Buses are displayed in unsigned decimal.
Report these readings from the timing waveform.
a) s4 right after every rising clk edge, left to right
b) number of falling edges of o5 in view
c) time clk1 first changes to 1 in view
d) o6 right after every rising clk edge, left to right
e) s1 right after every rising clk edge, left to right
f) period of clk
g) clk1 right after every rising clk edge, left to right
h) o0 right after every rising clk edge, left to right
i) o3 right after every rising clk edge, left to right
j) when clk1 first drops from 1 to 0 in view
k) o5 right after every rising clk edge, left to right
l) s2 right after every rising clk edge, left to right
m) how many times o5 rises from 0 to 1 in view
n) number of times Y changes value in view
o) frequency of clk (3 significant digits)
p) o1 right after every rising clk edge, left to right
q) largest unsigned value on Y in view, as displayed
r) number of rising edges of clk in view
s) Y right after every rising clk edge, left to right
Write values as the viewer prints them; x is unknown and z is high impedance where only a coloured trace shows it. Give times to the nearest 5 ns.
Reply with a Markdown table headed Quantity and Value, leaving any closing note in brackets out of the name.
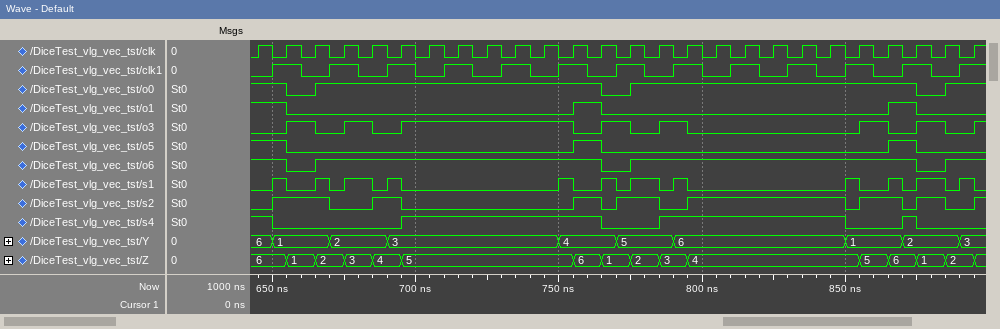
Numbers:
| Quantity | Value |
|---|---|
| s4 right after every rising clk edge, left to right | 1 0 0 0 0 1 1 1 1 1 1 1 0 0 1 1 1 1 1 1 1 0 0 0 0 0 |
| number of falling edges of o5 in view | 3 |
| time clk1 first changes to 1 in view | 650 ns |
| o6 right after every rising clk edge, left to right | 1 0 1 1 1 1 1 1 1 1 1 1 0 1 1 1 1 1 1 1 1 1 1 0 1 1 |
| s1 right after every rising clk edge, left to right | 0 0 1 1 0 0 0 0 0 0 0 0 1 1 0 0 0 0 0 0 0 0 1 1 0 0 |
| period of clk | 10 ns |
| clk1 right after every rising clk edge, left to right | 0 1 0 1 0 1 0 1 0 1 0 1 0 1 0 1 0 1 0 1 0 1 0 1 0 1 |
| o0 right after every rising clk edge, left to right | 1 0 1 1 1 1 1 1 1 1 1 1 0 1 1 1 1 1 1 1 1 1 1 0 1 1 |
| o3 right after every rising clk edge, left to right | 0 1 0 1 0 1 1 1 1 1 1 0 1 0 1 0 0 0 0 0 0 1 0 1 0 1 |
| when clk1 first drops from 1 to 0 in view | 660 ns |
| o5 right after every rising clk edge, left to right | 1 0 0 0 0 0 0 0 0 0 0 1 0 0 0 0 0 0 0 0 0 0 1 0 0 0 |
| s2 right after every rising clk edge, left to right | 0 1 1 0 1 0 0 0 0 0 0 1 0 1 0 1 1 1 1 1 1 1 1 1 0 1 |
| how many times o5 rises from 0 to 1 in view | 2 |
| number of times Y changes value in view | 9 |
| frequency of clk | 100 MHz |
| o1 right after every rising clk edge, left to right | 1 0 0 0 0 0 0 0 0 0 0 1 0 0 0 0 0 0 0 0 0 0 1 0 0 0 |
| largest unsigned value on Y in view, as displayed | 6 |
| number of rising edges of clk in view | 26 |
| Y right after every rising clk edge, left to right | 6, 1, 1, 2, 2, 3, 3, 3, 3, 3, 3, 4, 4, 5, 5, 6, 6, 6, 6, 6, 6, 1, 1, 2, 2, 3 |
